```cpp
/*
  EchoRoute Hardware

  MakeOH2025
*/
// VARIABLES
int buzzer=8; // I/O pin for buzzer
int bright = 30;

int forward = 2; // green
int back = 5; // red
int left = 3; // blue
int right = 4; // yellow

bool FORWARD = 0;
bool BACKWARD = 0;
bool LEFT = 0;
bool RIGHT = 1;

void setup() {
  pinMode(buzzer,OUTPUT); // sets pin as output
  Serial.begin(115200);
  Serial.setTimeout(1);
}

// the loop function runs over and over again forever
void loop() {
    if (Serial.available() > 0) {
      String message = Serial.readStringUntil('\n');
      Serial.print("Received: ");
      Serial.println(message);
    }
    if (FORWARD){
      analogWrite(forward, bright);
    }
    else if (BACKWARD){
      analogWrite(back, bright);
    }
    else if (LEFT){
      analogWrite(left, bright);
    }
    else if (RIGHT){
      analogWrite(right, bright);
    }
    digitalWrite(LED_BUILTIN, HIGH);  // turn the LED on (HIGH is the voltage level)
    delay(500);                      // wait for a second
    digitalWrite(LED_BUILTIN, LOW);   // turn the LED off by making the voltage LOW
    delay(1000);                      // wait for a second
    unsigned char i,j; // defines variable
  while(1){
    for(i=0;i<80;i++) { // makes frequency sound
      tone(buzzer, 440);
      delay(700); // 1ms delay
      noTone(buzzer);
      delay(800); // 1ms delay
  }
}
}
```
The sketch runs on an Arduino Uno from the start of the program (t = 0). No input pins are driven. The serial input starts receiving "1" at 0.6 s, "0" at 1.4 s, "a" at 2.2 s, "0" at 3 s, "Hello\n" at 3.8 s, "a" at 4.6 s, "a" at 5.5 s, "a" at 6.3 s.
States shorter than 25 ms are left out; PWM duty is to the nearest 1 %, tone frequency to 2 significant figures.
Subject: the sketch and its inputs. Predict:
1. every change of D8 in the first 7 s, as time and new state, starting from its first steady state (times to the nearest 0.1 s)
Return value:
0 s low; 1.5 s tone 440 Hz; 2.2 s low; 3 s tone 440 Hz; 3.7 s low; 4.5 s tone 440 Hz; 5.2 s low; 6 s tone 440 Hz; 6.7 s low
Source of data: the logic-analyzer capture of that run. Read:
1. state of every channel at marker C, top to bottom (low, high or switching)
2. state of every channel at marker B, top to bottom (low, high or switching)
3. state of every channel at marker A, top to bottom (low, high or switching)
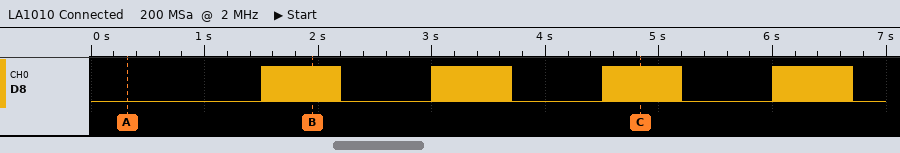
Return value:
D8 switching
D8 switching
D8 low
